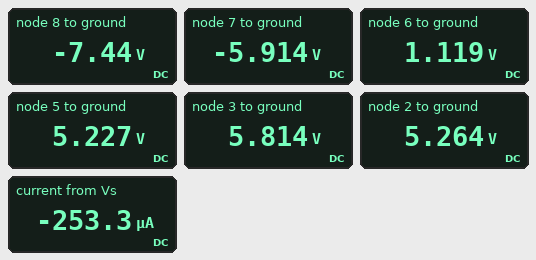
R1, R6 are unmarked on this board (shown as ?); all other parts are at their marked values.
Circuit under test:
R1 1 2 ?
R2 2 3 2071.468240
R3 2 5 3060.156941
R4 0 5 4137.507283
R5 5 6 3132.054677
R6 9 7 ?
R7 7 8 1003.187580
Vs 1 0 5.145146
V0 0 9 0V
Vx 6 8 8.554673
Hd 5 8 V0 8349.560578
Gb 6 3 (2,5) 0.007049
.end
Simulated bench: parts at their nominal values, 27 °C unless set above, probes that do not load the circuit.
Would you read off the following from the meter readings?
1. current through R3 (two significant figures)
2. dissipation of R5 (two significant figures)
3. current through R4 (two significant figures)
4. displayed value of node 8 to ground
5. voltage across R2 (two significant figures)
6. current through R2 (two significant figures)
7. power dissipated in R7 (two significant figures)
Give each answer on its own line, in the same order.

12 µA
5.4 mW
1.3 mA
-7.44 V
550 mV
270 µA
2.3 mW
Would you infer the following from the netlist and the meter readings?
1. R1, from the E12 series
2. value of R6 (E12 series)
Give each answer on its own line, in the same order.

470 Ω
3.9 kΩ
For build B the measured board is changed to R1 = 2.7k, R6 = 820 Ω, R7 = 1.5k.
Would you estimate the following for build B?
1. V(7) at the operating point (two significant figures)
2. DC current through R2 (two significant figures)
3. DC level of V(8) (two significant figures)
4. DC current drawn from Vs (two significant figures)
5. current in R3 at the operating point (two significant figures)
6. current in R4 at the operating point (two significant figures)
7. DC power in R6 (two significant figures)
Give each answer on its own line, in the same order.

-590 mV
340 µA
-1.7 V
330 µA
16 µA
1.0 mA
420 µW
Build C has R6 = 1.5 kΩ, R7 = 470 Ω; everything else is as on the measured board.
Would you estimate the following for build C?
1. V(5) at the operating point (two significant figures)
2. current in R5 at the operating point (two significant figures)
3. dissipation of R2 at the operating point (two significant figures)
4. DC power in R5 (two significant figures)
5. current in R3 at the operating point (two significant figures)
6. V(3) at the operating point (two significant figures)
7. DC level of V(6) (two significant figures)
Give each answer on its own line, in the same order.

5.0 V
640 µA
410 µW
1.3 mW
21 µA
4.0 V
7.0 V
